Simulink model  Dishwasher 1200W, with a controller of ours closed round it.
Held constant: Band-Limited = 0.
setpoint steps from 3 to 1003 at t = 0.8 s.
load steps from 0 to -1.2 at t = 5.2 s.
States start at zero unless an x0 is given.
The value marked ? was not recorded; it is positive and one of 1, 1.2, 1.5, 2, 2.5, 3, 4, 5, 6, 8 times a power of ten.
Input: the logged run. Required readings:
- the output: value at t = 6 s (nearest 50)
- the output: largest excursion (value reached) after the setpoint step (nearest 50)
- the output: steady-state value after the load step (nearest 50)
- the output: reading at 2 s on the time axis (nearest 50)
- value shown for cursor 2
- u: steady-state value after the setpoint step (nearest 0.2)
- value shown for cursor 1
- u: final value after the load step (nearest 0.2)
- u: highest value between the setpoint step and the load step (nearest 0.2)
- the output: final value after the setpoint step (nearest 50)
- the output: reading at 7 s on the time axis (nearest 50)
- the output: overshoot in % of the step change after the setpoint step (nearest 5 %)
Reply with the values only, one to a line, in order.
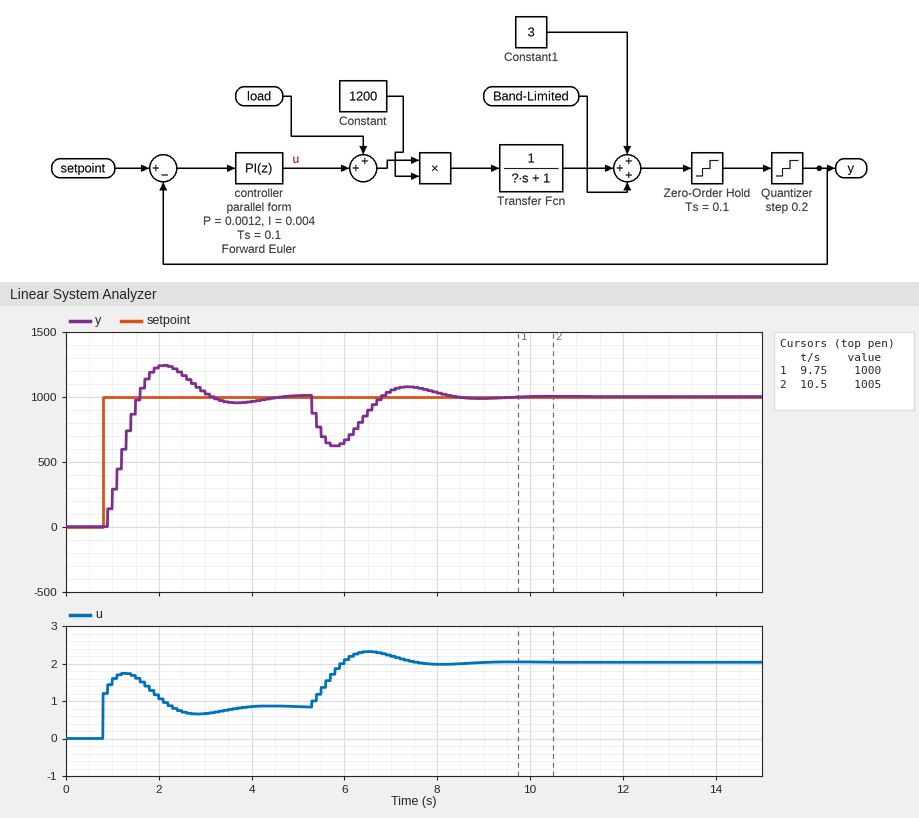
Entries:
650
1250
1000
1250
1005
0.8
1000
2.0
1.8
1000
1050
25 %
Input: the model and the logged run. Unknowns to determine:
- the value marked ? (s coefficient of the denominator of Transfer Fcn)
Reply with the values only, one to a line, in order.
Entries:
1
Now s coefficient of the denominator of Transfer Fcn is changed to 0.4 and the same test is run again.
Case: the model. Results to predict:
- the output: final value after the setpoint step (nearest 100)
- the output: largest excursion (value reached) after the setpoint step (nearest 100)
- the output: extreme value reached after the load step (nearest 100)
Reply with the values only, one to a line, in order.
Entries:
1000
1100
500
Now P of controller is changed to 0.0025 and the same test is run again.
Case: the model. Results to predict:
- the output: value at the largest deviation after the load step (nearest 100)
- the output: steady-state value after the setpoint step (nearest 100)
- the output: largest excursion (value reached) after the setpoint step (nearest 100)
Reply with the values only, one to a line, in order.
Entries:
700
1000
1100
